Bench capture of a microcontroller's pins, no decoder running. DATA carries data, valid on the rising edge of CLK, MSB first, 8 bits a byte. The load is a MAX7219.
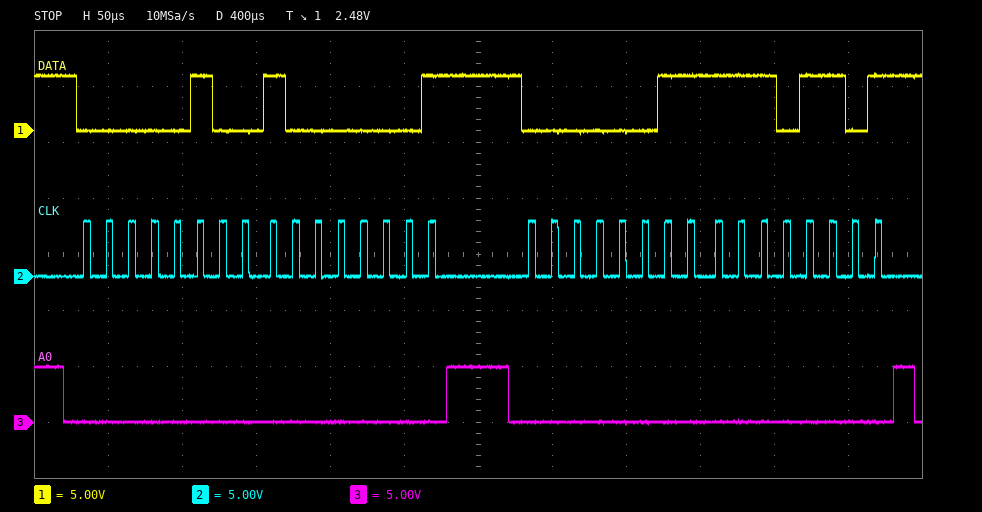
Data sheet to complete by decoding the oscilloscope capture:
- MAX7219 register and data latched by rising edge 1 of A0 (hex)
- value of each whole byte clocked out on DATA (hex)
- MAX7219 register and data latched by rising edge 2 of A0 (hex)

register 0x4, data 0x81
0x04 0x81 0x03 0xED
register 0x3, data 0xED
